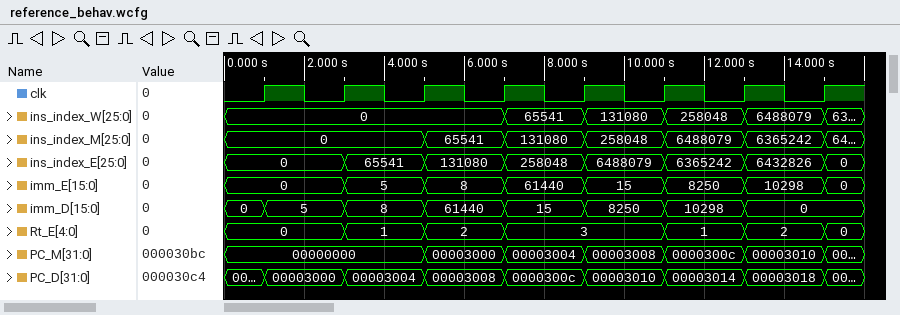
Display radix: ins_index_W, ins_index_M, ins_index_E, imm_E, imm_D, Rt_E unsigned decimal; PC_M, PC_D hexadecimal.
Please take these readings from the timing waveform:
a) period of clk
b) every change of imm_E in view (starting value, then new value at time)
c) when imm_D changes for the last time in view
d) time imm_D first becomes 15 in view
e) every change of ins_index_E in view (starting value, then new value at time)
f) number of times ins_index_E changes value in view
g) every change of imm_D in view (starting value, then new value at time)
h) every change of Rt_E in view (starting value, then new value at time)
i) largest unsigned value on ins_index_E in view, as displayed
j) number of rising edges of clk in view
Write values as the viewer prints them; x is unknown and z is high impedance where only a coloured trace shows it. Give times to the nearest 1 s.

2 s
0, 5 at 3 s, 8 at 5 s, 61440 at 7 s, 15 at 9 s, 8250 at 11 s, 10298 at 13 s, 0 at 15 s
13 s
7 s
0, 65541 at 3 s, 131080 at 5 s, 258048 at 7 s, 6488079 at 9 s, 6365242 at 11 s, 6432826 at 13 s, 0 at 15 s
7
0, 5 at 1 s, 8 at 3 s, 61440 at 5 s, 15 at 7 s, 8250 at 9 s, 10298 at 11 s, 0 at 13 s
0, 1 at 3 s, 2 at 5 s, 3 at 7 s, 1 at 11 s, 2 at 13 s, 0 at 15 s
6488079
8
